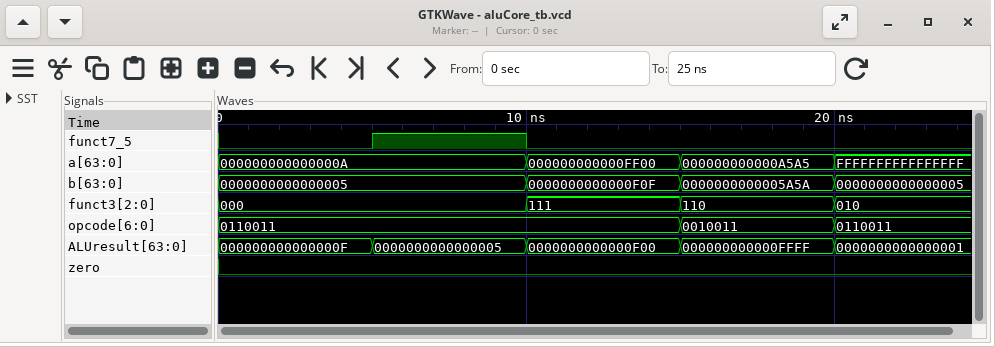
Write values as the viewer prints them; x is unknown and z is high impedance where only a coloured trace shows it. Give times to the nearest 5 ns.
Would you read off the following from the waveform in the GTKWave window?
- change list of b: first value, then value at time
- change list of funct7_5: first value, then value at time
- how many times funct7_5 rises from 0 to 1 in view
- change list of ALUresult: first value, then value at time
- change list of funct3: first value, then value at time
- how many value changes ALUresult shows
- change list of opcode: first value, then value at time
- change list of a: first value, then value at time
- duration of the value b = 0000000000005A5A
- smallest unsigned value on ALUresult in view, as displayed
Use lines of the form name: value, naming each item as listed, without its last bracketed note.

change list of b: first value, then value at time: 0000000000000005, 0000000000000F0F at 10 ns, 0000000000005A5A at 15 ns, 0000000000000005 at 20 ns
change list of funct7_5: first value, then value at time: 0, 1 at 5 ns, 0 at 10 ns
how many times funct7_5 rises from 0 to 1 in view: 1
change list of ALUresult: first value, then value at time: 000000000000000F, 0000000000000005 at 5 ns, 0000000000000F00 at 10 ns, 000000000000FFFF at 15 ns, 0000000000000001 at 20 ns
change list of funct3: first value, then value at time: 000, 111 at 10 ns, 110 at 15 ns, 010 at 20 ns
how many value changes ALUresult shows: 4
change list of opcode: first value, then value at time: 0110011, 0010011 at 15 ns, 0110011 at 20 ns
change list of a: first value, then value at time: 000000000000000A, 000000000000FF00 at 10 ns, 000000000000A5A5 at 15 ns, FFFFFFFFFFFFFFFF at 20 ns
duration of the value b = 0000000000005A5A: 5 ns
smallest unsigned value on ALUresult in view, as displayed: 0000000000000001
